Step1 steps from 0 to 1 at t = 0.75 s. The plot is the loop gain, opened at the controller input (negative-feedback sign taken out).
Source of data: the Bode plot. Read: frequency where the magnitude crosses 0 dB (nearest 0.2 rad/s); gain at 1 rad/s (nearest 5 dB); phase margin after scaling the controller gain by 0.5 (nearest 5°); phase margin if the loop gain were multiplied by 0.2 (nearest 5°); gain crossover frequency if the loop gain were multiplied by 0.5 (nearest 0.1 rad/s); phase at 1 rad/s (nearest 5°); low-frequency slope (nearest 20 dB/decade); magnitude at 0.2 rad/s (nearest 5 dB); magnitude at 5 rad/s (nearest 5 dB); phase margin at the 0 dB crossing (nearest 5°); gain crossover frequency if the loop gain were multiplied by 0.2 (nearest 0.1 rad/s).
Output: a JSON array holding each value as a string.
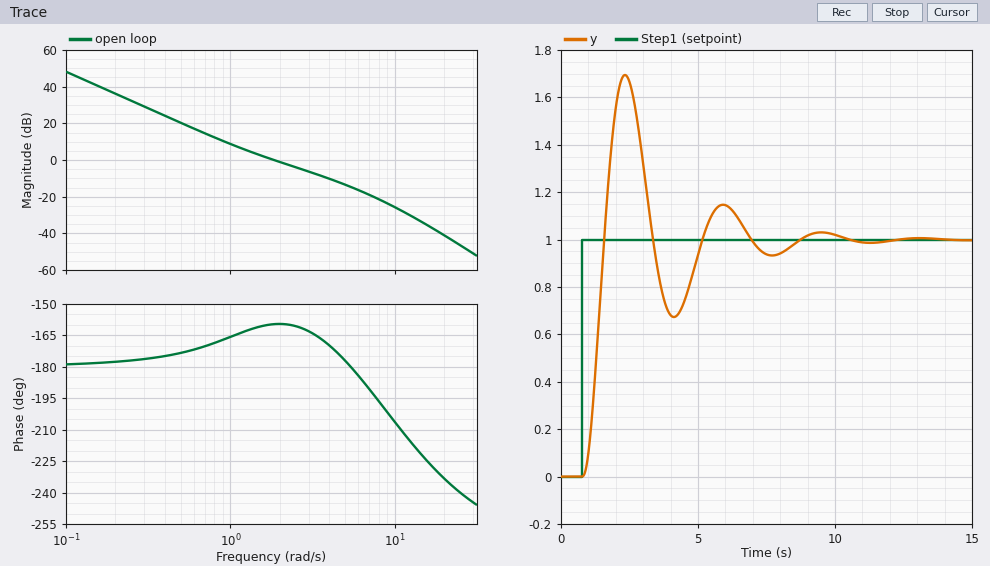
["1.8 rad/s", "10 dB", "15°", "10°", "1.2 rad/s", "-165°", "-40 dB/decade", "35 dB", "-15 dB", "20°", "0.7 rad/s"]
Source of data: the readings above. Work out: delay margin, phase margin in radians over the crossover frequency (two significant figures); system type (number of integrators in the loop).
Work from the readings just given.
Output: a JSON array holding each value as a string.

["0.19 s", "2"]
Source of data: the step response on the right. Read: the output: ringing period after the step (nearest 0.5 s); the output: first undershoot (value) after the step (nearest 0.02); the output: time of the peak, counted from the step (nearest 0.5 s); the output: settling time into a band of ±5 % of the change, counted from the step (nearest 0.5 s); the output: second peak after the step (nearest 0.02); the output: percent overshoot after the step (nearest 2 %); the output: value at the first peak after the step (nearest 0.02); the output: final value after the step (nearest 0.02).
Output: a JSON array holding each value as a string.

["3.5 s", "0.68", "1.5 s", "7.5 s", "1.14", "70 %", "1.70", "1.00"]
